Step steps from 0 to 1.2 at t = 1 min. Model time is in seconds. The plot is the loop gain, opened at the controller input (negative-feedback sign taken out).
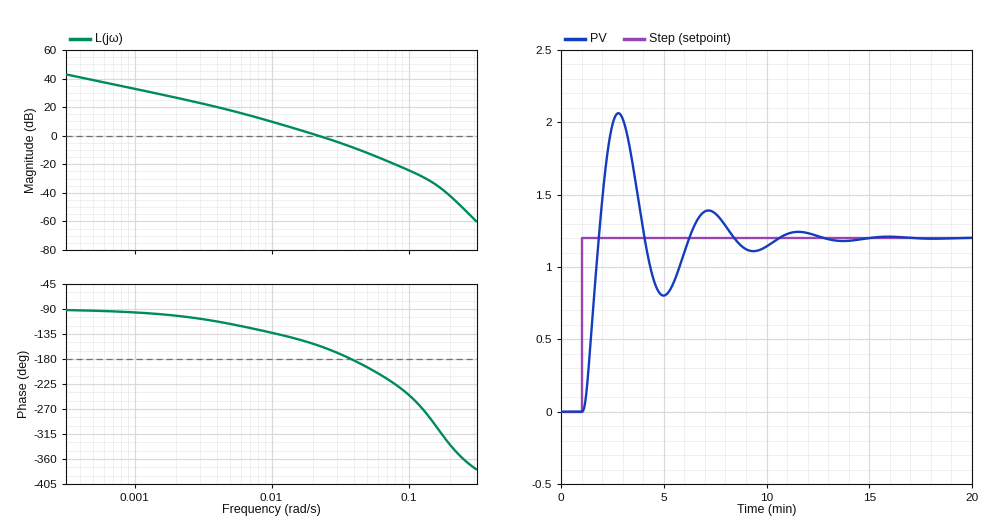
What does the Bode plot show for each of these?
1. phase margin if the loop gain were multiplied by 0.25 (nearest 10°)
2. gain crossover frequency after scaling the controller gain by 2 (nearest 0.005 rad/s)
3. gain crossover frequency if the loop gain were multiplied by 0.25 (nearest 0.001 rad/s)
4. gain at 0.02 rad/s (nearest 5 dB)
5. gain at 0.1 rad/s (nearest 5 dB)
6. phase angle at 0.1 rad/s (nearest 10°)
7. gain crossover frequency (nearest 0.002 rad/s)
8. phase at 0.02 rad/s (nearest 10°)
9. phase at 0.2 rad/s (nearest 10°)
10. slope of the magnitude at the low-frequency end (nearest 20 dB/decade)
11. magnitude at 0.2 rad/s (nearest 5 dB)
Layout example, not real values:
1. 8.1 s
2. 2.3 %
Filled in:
1. 50°
2. 0.035 rad/s
3. 0.008 rad/s
4. 0 dB
5. -25 dB
6. -240°
7. 0.022 rad/s
8. -150°
9. -330°
10. -20 dB/decade
11. -40 dB
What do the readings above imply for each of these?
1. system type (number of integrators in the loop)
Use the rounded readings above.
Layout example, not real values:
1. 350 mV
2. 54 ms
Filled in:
1. 1
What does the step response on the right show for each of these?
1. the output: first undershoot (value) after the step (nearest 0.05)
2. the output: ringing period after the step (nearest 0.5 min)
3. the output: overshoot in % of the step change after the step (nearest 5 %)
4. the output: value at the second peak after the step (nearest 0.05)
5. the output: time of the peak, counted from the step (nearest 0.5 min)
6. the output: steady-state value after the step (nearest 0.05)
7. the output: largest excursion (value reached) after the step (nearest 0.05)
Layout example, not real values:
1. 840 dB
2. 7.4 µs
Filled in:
1. 0.80
2. 4.5 min
3. 70 %
4. 1.40
5. 2.0 min
6. 1.20
7. 2.05
